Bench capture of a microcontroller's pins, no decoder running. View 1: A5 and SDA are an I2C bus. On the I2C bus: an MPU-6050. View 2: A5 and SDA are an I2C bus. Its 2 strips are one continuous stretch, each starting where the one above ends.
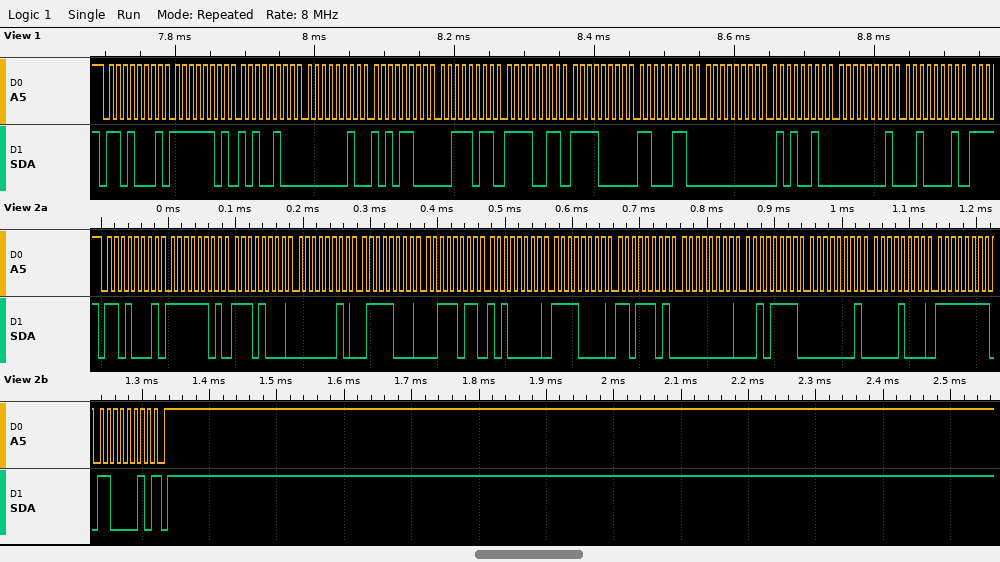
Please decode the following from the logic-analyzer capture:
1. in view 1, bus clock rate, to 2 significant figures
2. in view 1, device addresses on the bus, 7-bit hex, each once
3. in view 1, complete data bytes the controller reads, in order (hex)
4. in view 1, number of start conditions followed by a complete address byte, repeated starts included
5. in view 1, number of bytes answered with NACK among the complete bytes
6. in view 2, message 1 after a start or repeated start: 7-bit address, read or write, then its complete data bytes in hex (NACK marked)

100 kHz
0x68
FD A4 02 AC 3B F3 F0 C6 00 52 01 21
1
0
0x68 read: FD E8 02 78 3B A0 F0 DD 00 2F 01 08 FF C2 NACK
